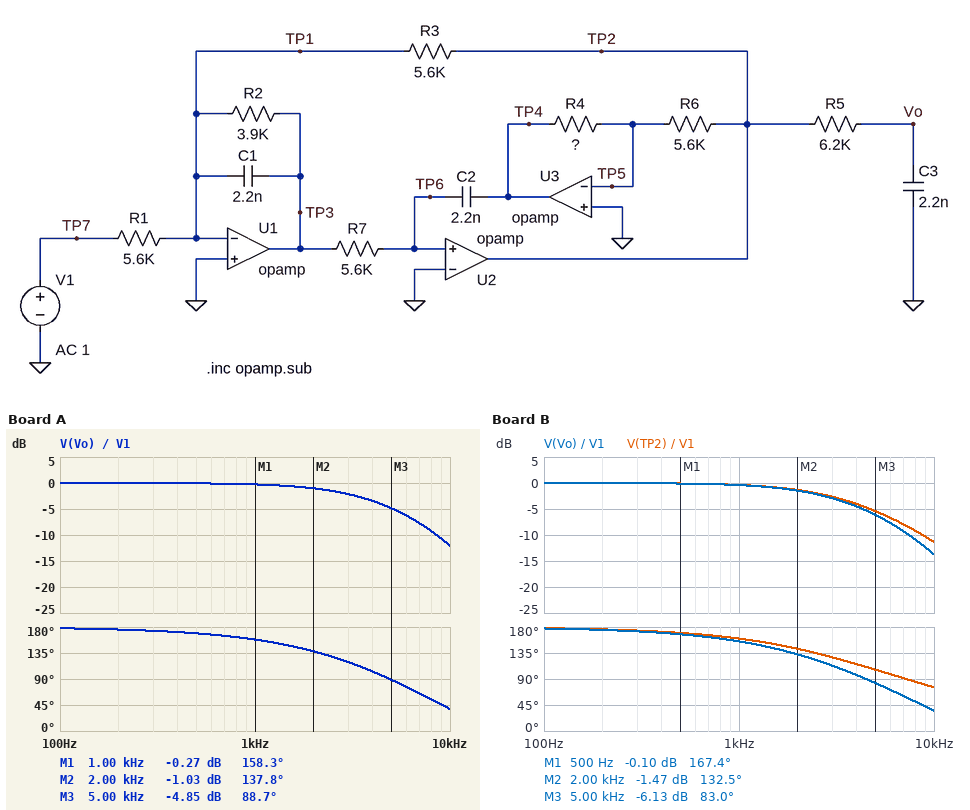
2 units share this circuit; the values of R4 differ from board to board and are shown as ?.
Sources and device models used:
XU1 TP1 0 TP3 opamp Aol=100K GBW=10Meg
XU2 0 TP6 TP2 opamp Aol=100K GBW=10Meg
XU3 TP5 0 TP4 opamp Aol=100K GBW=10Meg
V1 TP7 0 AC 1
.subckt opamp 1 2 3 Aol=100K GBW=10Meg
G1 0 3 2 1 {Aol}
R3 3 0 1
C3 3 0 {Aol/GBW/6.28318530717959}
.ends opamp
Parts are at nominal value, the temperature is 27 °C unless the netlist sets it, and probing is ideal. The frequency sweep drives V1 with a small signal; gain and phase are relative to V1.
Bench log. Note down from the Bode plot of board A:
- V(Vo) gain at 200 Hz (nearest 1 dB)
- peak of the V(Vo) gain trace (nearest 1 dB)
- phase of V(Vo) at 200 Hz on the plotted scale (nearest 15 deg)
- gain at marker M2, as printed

0 dB
0 dB
180 deg
-1.03 dB
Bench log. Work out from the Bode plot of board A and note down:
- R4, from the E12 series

15 kΩ
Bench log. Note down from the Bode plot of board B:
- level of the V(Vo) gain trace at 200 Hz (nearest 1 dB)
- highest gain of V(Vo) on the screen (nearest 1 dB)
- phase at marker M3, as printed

0 dB
0 dB
83.0 deg
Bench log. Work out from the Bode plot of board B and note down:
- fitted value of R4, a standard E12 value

18 kΩ
